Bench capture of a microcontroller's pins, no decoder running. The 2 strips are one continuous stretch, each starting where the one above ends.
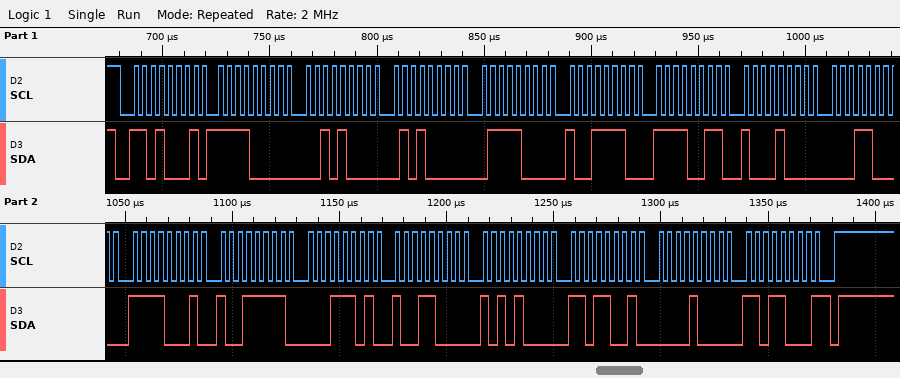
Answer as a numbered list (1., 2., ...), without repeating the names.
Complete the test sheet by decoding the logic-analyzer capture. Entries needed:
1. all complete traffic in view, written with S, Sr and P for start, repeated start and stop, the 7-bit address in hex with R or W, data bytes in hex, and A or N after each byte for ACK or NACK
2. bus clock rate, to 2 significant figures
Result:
1. S 68R A F0 A 28 A 50 A 78 A 9E A F3 A 88 A 18 A F1 A 9F A 1D A 98 A A8 A D9 A 08 A D8 N P
2. 250 kHz
